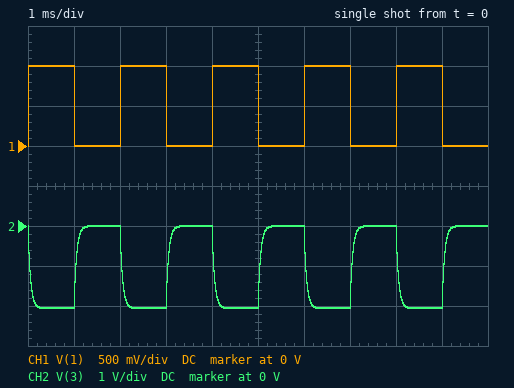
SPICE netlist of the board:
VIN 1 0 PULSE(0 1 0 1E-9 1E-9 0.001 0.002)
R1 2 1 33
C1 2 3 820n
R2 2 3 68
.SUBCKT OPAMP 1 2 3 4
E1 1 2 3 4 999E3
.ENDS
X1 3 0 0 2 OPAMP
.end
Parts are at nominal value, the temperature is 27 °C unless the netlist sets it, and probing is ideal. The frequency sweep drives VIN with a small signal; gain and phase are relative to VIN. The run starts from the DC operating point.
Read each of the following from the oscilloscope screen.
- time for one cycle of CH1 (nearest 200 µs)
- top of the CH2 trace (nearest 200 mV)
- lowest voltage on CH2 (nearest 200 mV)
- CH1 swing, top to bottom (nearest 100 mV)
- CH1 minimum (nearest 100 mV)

2.0 ms
0 V
-2.0 V
1.0 V
0 V
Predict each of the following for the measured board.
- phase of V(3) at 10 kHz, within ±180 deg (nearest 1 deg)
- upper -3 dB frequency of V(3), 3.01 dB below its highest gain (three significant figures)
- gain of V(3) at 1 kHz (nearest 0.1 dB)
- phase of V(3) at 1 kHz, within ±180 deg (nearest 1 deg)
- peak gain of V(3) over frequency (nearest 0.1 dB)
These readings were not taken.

106 deg
2.85 kHz
5.8 dB
161 deg
6.3 dB
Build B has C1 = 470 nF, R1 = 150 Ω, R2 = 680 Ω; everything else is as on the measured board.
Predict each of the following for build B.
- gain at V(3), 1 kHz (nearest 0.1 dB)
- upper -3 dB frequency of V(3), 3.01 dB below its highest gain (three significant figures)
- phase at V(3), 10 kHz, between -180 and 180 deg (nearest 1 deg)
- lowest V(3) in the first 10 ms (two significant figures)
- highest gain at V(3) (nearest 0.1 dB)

6.1 dB
498 Hz
93 deg
-4.3 V
13.1 dB
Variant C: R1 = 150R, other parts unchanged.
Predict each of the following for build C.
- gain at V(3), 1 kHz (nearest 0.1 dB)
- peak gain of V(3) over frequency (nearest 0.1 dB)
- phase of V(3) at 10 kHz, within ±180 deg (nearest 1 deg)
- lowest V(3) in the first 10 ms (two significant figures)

-7.4 dB
-6.9 dB
106 deg
-450 mV
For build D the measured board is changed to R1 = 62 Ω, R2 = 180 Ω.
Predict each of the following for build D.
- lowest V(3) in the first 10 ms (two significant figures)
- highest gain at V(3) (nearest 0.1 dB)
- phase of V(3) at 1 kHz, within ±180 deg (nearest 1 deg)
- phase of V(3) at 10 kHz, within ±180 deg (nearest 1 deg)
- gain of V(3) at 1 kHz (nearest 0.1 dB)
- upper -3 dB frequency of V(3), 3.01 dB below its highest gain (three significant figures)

-2.9 V
9.3 dB
137 deg
96 deg
6.6 dB
1.08 kHz
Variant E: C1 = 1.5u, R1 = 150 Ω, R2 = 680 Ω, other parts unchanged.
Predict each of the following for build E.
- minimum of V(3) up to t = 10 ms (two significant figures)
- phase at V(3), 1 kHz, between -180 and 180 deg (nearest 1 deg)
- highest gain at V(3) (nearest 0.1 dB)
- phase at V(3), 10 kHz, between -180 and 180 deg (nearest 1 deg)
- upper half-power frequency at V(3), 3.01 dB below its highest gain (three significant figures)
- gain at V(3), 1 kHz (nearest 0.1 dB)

-3.3 V
99 deg
13.1 dB
91 deg
156 Hz
-3.1 dB
